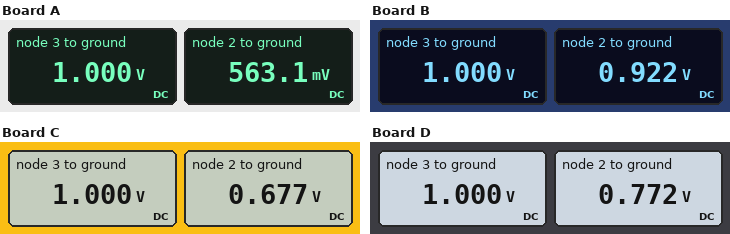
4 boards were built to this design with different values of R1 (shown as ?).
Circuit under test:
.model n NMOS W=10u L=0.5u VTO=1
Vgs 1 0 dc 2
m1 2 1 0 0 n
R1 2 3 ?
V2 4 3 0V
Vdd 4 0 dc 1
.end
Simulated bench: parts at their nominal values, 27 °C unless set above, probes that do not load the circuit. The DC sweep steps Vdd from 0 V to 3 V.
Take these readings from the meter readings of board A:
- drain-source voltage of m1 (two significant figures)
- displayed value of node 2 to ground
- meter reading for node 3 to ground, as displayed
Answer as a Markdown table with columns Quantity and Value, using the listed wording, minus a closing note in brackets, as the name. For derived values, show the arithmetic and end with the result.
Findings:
| Quantity | Value |
|---|---|
| drain-source voltage of m1 | 563.1 mV = 560 mV |
| displayed value of node 2 to ground | 563.1 mV |
| meter reading for node 3 to ground, as displayed | 1.000 V |
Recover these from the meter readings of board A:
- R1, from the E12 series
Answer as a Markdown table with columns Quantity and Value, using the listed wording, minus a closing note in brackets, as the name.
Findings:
| Quantity | Value |
|---|---|
| R1, from the E12 series | 2.7 kΩ |
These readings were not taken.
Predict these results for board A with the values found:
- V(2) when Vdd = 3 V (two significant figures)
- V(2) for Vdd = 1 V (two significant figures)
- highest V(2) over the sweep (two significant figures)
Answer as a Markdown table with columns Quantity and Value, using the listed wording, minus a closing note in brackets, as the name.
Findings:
| Quantity | Value |
|---|---|
| V(2) when Vdd = 3 V | 2.5 V |
| V(2) for Vdd = 1 V | 560 mV |
| highest V(2) over the sweep | 2.5 V |
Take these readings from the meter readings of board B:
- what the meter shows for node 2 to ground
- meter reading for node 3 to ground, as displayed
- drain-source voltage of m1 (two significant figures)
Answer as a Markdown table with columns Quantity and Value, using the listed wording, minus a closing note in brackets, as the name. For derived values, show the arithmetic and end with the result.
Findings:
| Quantity | Value |
|---|---|
| what the meter shows for node 2 to ground | 0.922 V |
| meter reading for node 3 to ground, as displayed | 1.000 V |
| drain-source voltage of m1 | 922 mV = 920 mV |
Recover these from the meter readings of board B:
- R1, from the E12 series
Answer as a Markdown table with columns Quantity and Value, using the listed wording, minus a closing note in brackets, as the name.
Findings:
| Quantity | Value |
|---|---|
| R1, from the E12 series | 390 Ω |
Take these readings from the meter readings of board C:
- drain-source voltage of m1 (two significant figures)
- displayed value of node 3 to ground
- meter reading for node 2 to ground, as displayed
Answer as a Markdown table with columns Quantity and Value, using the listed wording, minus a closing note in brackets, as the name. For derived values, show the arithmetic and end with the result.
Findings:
| Quantity | Value |
|---|---|
| drain-source voltage of m1 | 677 mV = 680 mV |
| displayed value of node 3 to ground | 1.000 V |
| meter reading for node 2 to ground, as displayed | 0.677 V |
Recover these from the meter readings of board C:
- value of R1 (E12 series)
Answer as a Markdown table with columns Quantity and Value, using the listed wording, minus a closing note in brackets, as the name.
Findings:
| Quantity | Value |
|---|---|
| value of R1 | 1.8 kΩ |
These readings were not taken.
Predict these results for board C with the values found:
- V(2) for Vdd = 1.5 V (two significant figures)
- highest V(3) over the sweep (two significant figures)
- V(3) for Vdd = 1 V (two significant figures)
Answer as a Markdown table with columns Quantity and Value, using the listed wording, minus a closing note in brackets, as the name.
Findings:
| Quantity | Value |
|---|---|
| V(2) for Vdd = 1.5 V | 1.1 V |
| highest V(3) over the sweep | 3.0 V |
| V(3) for Vdd = 1 V | 1.0 V |
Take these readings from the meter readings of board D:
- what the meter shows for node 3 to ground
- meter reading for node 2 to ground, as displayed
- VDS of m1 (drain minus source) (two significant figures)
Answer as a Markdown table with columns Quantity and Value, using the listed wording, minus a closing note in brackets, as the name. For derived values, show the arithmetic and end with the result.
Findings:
| Quantity | Value |
|---|---|
| what the meter shows for node 3 to ground | 1.000 V |
| meter reading for node 2 to ground, as displayed | 0.772 V |
| VDS of m1 (drain minus source) | 772 mV = 770 mV |
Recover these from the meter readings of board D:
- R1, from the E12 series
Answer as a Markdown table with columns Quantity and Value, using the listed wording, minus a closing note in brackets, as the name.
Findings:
| Quantity | Value |
|---|---|
| R1, from the E12 series | 1.2 kΩ |
